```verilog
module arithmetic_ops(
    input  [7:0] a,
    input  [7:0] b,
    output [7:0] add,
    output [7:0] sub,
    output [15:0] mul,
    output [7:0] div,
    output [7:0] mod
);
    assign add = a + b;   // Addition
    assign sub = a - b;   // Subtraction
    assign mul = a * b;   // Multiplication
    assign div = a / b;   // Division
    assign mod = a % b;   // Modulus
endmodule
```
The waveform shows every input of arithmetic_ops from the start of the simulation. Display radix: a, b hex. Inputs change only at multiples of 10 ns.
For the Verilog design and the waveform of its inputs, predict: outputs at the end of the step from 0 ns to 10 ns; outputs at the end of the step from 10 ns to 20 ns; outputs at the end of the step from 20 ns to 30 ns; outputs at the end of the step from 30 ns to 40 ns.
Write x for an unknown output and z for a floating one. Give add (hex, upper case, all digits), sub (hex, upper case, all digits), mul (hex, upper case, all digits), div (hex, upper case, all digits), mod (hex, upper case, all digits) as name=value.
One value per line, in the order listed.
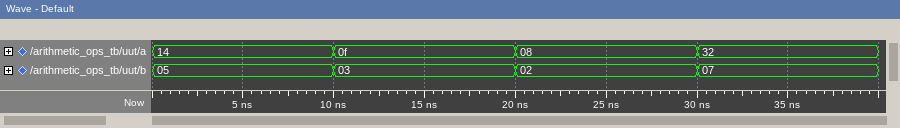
add=19, sub=0F, mul=0064, div=04, mod=00
add=12, sub=0C, mul=002D, div=05, mod=00
add=0A, sub=06, mul=0010, div=04, mod=00
add=39, sub=2B, mul=015E, div=07, mod=01
